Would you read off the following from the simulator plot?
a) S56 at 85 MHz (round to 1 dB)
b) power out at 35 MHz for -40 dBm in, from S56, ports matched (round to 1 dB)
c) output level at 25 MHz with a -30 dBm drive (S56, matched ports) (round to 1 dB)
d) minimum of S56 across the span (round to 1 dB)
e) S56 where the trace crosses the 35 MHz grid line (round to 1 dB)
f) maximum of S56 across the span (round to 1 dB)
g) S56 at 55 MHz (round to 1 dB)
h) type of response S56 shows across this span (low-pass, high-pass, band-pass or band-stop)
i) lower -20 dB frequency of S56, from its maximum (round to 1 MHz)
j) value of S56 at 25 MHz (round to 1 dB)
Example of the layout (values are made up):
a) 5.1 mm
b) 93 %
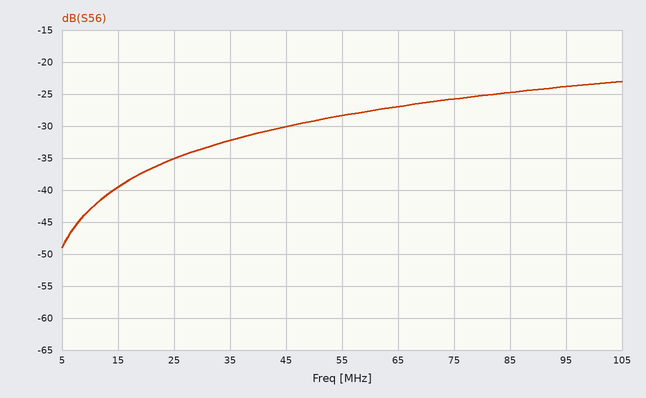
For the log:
a) -25 dB
b) -72 dBm
c) -65 dBm
d) -49 dB
e) -32 dB
f) -23 dB
g) -28 dB
h) high-pass
i) 10 MHz
j) -35 dB
